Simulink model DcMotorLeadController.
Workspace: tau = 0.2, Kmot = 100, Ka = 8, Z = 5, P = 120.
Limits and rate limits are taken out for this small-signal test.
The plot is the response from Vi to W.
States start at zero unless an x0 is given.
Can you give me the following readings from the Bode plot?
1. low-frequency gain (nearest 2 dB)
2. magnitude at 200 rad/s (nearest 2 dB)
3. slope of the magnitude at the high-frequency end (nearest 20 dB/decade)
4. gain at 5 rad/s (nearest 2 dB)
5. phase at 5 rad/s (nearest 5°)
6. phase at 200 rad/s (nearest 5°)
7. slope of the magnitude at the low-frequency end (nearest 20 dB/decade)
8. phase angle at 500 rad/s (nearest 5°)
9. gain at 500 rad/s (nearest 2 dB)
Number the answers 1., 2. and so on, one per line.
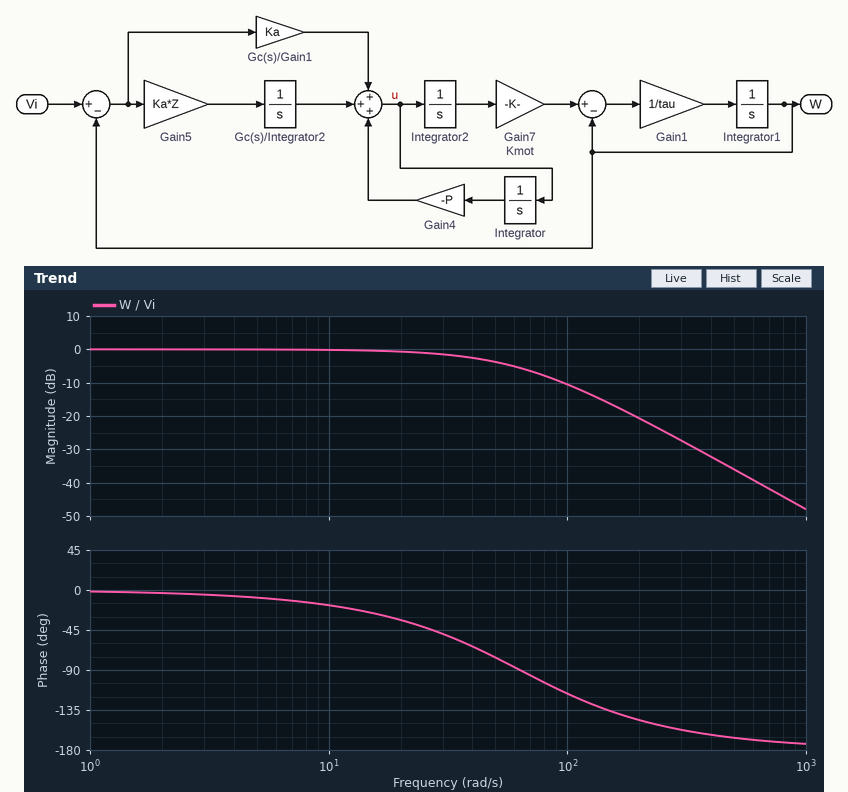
1. 0 dB
2. -20 dB
3. -40 dB/decade
4. 0 dB
5. -10°
6. -145°
7. 0 dB/decade
8. -165°
9. -36 dB
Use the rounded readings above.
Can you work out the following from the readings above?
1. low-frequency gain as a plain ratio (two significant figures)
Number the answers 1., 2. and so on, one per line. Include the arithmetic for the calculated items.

1. 10^(0 / 20) = 1.0
